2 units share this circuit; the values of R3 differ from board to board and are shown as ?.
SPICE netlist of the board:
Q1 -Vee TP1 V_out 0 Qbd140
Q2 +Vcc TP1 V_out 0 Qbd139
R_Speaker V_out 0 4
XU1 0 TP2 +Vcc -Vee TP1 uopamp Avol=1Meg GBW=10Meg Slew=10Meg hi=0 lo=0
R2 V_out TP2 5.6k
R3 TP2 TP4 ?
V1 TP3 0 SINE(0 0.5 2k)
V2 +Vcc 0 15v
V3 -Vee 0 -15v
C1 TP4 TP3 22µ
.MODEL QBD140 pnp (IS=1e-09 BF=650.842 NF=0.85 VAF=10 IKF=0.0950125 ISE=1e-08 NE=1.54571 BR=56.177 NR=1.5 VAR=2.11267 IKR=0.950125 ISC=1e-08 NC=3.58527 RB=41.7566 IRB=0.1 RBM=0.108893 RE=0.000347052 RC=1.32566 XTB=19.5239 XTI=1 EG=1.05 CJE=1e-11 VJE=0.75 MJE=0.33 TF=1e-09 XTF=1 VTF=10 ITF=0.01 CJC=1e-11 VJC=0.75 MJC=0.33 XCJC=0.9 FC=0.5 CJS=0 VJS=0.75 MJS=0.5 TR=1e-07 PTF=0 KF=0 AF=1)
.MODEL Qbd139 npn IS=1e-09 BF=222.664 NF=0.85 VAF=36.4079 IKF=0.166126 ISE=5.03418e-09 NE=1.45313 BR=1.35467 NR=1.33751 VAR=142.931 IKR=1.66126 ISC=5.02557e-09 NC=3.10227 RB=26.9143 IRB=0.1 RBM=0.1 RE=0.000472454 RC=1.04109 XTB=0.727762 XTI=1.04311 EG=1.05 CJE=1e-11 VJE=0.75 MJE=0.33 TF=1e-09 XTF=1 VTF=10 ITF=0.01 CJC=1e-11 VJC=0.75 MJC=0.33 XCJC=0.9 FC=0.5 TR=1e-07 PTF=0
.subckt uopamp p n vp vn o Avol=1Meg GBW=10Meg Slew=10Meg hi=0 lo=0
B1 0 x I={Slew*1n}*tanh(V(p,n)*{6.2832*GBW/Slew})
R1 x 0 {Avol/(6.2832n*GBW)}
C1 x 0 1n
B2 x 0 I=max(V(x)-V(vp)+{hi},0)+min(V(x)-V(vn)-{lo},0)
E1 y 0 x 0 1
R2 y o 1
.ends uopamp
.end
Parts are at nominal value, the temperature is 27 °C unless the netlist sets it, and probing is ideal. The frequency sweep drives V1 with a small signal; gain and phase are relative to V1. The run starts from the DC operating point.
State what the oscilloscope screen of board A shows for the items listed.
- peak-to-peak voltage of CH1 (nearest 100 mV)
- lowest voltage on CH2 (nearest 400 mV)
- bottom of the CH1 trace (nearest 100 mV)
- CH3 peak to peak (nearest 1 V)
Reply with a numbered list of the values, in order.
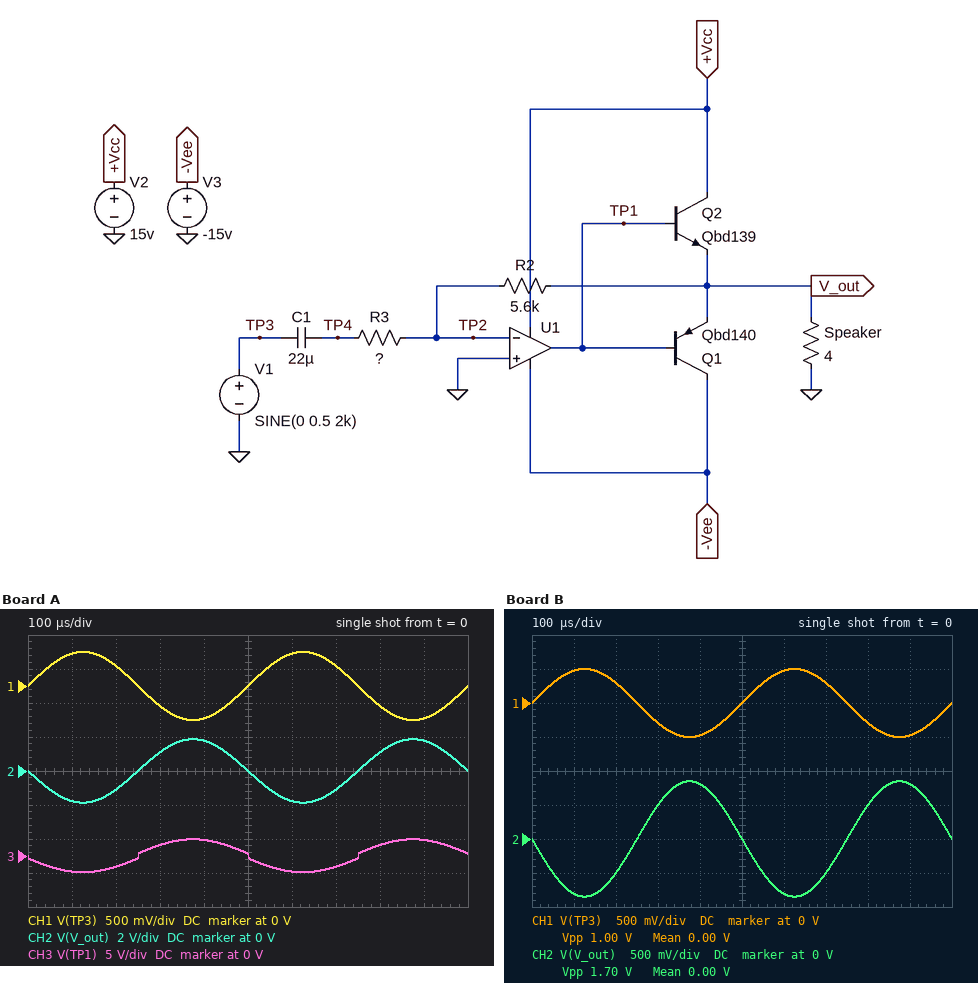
1. 1.0 V
2. -2.0 V
3. -500 mV
4. 5 V
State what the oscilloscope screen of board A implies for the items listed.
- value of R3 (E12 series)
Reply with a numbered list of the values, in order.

1. 1.5 kΩ
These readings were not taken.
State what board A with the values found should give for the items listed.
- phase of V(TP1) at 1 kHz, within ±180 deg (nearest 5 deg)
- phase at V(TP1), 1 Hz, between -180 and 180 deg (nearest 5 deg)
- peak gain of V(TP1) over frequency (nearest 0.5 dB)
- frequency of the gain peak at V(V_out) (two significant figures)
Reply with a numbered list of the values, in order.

1. 90 deg
2. -115 deg
3. 114.0 dB
4. 5.7 Hz
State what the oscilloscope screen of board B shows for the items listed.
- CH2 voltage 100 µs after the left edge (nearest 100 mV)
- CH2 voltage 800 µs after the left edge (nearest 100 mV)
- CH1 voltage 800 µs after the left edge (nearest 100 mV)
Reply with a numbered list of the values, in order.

1. -800 mV
2. 500 mV
3. -300 mV
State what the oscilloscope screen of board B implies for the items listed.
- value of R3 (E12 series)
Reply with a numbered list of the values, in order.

1. 3.3 kΩ
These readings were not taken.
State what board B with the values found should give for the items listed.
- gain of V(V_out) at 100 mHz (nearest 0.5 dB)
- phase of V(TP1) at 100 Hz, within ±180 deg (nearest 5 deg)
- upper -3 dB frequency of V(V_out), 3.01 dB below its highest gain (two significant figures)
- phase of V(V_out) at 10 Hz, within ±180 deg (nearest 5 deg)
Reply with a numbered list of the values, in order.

1. -25.5 dB
2. 100 deg
3. 20 Hz
4. 160 deg
